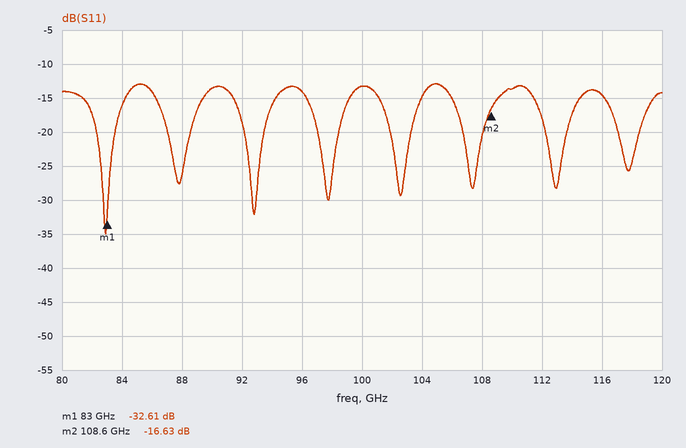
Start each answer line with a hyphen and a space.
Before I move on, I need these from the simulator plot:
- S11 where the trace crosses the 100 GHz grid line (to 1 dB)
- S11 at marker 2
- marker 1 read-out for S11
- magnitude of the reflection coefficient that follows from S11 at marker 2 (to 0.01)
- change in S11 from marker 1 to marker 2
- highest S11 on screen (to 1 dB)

- -13 dB
- -16.63 dB
- -32.61 dB
- 0.15
- 15.98 dB
- -13 dB
